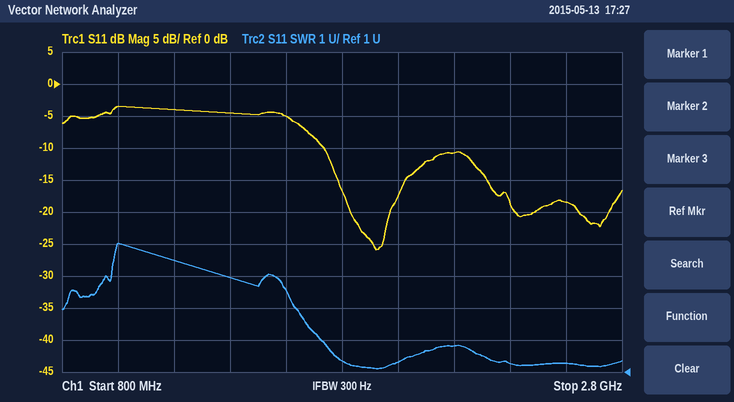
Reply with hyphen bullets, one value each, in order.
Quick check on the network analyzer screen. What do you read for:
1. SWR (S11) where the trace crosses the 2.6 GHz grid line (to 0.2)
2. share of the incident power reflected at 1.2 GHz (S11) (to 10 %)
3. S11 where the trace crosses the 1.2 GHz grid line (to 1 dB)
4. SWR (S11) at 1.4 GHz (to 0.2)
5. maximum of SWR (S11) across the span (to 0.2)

- 1.2
- 40 %
- -4 dB
- 4.0
- 5.0
